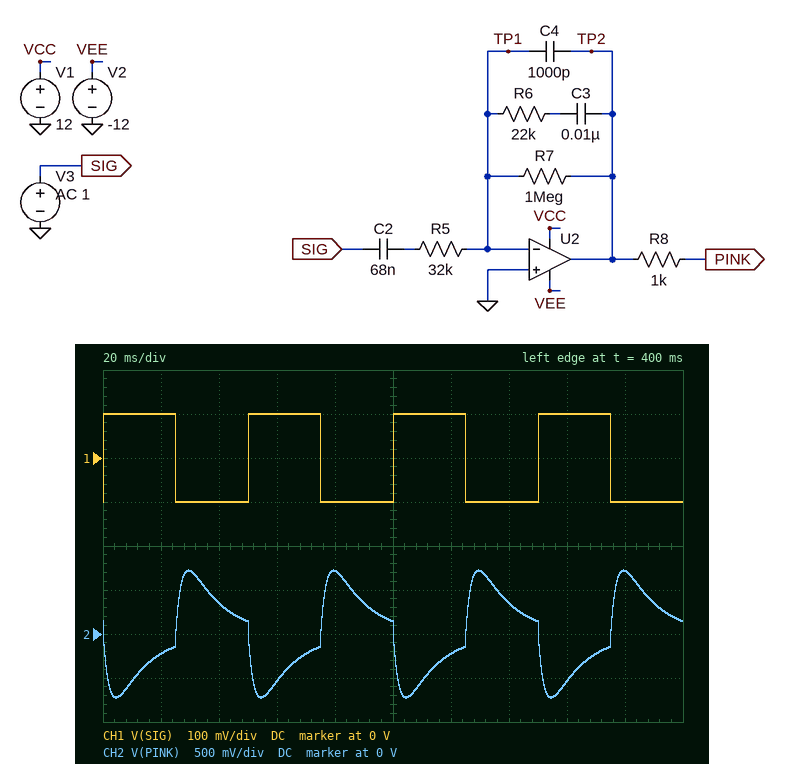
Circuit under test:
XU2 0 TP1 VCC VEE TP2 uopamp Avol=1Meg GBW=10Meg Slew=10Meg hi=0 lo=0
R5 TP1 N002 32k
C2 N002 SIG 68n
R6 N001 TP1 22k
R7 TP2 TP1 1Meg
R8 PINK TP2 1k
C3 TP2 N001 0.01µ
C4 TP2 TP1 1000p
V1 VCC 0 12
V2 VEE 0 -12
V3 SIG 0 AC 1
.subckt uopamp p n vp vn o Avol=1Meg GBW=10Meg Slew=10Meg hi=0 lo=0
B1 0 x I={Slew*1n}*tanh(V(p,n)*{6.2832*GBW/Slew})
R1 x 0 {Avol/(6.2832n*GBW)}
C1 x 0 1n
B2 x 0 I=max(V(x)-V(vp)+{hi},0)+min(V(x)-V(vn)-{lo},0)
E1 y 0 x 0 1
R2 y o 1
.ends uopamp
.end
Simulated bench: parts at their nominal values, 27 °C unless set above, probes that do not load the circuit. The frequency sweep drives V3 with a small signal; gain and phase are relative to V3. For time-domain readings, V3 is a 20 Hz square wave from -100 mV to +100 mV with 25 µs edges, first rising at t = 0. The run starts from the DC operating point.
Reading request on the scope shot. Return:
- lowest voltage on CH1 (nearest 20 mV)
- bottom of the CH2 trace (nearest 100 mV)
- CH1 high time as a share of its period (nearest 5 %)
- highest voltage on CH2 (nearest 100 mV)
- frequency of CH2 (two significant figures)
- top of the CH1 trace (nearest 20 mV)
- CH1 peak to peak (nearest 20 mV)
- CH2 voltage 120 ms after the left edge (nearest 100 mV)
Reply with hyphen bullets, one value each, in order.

- -100 mV
- -700 mV
- 50 %
- 700 mV
- 20 Hz
- 100 mV
- 200 mV
- -200 mV
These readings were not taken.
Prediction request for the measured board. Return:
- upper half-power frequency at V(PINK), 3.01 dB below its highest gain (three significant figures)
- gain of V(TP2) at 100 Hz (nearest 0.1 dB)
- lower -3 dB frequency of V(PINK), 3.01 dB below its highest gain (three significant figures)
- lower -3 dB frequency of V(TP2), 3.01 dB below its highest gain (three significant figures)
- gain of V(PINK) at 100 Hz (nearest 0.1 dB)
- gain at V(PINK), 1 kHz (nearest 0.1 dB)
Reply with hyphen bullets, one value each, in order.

- 99.3 Hz
- 11.1 dB
- 10.6 Hz
- 10.6 Hz
- 11.1 dB
- -2.5 dB
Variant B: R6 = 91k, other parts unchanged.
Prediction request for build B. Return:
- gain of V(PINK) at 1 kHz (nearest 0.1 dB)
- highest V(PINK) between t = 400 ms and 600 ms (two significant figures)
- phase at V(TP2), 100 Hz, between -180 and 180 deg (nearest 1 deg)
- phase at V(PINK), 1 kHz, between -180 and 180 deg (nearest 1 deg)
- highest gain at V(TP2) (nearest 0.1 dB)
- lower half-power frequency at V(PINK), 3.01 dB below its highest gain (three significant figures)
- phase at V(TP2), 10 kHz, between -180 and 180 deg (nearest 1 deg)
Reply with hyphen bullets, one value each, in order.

- 6.8 dB
- 700 mV
- 161 deg
- 149 deg
- 13.9 dB
- 10.4 Hz
- 101 deg
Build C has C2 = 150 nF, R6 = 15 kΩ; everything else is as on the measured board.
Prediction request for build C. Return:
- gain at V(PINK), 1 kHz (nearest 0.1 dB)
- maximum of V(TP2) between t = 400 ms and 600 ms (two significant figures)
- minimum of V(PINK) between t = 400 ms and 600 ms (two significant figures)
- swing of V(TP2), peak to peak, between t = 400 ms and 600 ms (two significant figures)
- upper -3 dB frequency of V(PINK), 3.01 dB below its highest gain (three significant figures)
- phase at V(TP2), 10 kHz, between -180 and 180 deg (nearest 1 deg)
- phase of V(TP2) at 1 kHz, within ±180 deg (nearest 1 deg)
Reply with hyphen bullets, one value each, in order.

- -4.3 dB
- 1.2 V
- -1.2 V
- 2.4 V
- 56.0 Hz
- 134 deg
- 131 deg
